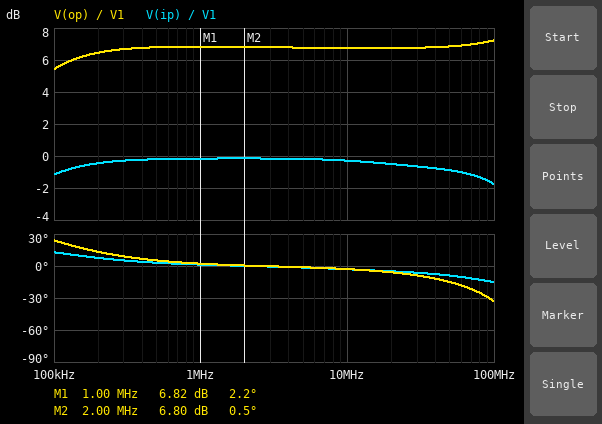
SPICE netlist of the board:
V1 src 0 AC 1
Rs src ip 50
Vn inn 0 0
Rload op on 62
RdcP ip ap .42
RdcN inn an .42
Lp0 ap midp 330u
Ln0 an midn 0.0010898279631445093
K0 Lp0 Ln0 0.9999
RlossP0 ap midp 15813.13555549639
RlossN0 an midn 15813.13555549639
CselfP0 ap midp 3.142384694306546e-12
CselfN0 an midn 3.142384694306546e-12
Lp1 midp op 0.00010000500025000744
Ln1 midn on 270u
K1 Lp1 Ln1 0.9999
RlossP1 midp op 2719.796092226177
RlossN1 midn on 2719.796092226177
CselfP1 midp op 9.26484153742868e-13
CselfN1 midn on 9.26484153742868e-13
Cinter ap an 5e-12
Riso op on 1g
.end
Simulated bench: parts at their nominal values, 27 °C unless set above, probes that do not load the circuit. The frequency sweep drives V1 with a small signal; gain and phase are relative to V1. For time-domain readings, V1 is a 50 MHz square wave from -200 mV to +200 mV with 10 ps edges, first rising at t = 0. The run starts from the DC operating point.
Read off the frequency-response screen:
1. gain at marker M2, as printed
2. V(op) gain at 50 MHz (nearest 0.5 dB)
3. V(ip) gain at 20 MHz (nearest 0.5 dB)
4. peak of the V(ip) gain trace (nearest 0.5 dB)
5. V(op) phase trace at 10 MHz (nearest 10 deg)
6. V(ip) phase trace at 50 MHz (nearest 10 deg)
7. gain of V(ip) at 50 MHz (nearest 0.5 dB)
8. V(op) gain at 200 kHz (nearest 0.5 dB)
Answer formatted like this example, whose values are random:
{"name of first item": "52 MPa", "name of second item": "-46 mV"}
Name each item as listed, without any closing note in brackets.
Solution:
{"gain at marker M2, as printed": "6.80 dB", "V(op) gain at 50 MHz": "7.0 dB", "V(ip) gain at 20 MHz": "-0.5 dB", "peak of the V(ip) gain trace": "0 dB", "V(op) phase trace at 10 MHz": "0 deg", "V(ip) phase trace at 50 MHz": "-10 deg", "gain of V(ip) at 50 MHz": "-1.0 dB", "V(op) gain at 200 kHz": "6.5 dB"}
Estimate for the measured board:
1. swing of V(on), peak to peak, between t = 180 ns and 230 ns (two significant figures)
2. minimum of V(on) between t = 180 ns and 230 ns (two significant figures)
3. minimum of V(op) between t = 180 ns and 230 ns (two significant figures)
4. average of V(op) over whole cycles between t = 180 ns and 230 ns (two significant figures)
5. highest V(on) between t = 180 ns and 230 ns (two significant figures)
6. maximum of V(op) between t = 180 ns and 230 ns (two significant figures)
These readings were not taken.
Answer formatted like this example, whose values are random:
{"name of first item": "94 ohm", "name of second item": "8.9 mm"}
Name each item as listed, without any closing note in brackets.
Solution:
{"swing of V(on), peak to peak, between t = 180 ns and 230 ns": "1.1 V", "minimum of V(on) between t = 180 ns and 230 ns": "-160 mV", "minimum of V(op) between t = 180 ns and 230 ns": "-280 mV", "average of V(op) over whole cycles between t = 180 ns and 230 ns": "300 mV", "highest V(on) between t = 180 ns and 230 ns": "960 mV", "maximum of V(op) between t = 180 ns and 230 ns": "890 mV"}
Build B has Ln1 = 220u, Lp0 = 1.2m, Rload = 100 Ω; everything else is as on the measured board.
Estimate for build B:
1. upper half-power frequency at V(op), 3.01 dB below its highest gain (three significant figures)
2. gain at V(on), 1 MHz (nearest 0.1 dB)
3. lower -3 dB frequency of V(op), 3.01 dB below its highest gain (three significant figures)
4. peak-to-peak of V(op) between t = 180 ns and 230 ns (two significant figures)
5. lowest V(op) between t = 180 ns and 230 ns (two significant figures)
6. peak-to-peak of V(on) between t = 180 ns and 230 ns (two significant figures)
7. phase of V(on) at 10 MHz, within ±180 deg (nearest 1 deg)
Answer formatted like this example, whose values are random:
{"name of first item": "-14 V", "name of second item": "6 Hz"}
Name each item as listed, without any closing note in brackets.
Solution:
{"upper half-power frequency at V(op), 3.01 dB below its highest gain": "102 MHz", "gain at V(on), 1 MHz": "-7.1 dB", "lower -3 dB frequency of V(op), 3.01 dB below its highest gain": "2.71 MHz", "peak-to-peak of V(op) between t = 180 ns and 230 ns": "900 mV", "lowest V(op) between t = 180 ns and 230 ns": "-490 mV", "peak-to-peak of V(on) between t = 180 ns and 230 ns": "770 mV", "phase of V(on) at 10 MHz, within ±180 deg": "9 deg"}
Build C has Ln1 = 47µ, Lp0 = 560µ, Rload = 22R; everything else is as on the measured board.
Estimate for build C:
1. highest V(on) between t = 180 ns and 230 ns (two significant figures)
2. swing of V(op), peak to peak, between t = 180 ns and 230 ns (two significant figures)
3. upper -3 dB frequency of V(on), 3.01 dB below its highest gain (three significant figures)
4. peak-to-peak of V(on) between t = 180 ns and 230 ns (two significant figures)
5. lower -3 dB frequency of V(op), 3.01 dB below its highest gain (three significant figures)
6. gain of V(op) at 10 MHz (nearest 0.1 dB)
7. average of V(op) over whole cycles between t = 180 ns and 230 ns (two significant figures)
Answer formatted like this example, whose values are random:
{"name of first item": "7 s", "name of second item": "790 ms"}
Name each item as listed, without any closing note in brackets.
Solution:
{"highest V(on) between t = 180 ns and 230 ns": "880 mV", "swing of V(op), peak to peak, between t = 180 ns and 230 ns": "740 mV", "upper -3 dB frequency of V(on), 3.01 dB below its highest gain": "13.3 MHz", "peak-to-peak of V(on) between t = 180 ns and 230 ns": "800 mV", "lower -3 dB frequency of V(op), 3.01 dB below its highest gain": "122 kHz", "gain of V(op) at 10 MHz": "7.4 dB", "average of V(op) over whole cycles between t = 180 ns and 230 ns": "430 mV"}
